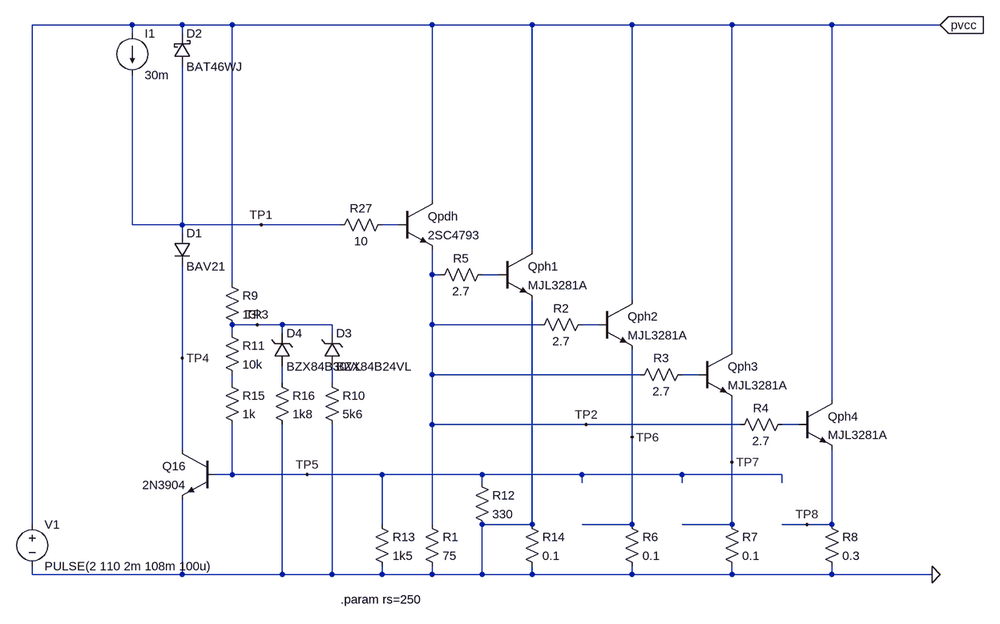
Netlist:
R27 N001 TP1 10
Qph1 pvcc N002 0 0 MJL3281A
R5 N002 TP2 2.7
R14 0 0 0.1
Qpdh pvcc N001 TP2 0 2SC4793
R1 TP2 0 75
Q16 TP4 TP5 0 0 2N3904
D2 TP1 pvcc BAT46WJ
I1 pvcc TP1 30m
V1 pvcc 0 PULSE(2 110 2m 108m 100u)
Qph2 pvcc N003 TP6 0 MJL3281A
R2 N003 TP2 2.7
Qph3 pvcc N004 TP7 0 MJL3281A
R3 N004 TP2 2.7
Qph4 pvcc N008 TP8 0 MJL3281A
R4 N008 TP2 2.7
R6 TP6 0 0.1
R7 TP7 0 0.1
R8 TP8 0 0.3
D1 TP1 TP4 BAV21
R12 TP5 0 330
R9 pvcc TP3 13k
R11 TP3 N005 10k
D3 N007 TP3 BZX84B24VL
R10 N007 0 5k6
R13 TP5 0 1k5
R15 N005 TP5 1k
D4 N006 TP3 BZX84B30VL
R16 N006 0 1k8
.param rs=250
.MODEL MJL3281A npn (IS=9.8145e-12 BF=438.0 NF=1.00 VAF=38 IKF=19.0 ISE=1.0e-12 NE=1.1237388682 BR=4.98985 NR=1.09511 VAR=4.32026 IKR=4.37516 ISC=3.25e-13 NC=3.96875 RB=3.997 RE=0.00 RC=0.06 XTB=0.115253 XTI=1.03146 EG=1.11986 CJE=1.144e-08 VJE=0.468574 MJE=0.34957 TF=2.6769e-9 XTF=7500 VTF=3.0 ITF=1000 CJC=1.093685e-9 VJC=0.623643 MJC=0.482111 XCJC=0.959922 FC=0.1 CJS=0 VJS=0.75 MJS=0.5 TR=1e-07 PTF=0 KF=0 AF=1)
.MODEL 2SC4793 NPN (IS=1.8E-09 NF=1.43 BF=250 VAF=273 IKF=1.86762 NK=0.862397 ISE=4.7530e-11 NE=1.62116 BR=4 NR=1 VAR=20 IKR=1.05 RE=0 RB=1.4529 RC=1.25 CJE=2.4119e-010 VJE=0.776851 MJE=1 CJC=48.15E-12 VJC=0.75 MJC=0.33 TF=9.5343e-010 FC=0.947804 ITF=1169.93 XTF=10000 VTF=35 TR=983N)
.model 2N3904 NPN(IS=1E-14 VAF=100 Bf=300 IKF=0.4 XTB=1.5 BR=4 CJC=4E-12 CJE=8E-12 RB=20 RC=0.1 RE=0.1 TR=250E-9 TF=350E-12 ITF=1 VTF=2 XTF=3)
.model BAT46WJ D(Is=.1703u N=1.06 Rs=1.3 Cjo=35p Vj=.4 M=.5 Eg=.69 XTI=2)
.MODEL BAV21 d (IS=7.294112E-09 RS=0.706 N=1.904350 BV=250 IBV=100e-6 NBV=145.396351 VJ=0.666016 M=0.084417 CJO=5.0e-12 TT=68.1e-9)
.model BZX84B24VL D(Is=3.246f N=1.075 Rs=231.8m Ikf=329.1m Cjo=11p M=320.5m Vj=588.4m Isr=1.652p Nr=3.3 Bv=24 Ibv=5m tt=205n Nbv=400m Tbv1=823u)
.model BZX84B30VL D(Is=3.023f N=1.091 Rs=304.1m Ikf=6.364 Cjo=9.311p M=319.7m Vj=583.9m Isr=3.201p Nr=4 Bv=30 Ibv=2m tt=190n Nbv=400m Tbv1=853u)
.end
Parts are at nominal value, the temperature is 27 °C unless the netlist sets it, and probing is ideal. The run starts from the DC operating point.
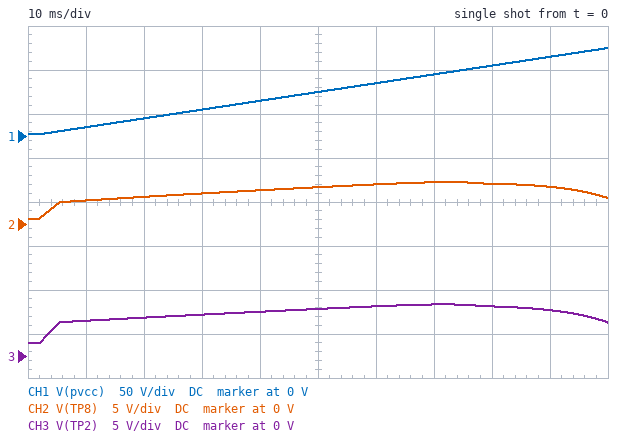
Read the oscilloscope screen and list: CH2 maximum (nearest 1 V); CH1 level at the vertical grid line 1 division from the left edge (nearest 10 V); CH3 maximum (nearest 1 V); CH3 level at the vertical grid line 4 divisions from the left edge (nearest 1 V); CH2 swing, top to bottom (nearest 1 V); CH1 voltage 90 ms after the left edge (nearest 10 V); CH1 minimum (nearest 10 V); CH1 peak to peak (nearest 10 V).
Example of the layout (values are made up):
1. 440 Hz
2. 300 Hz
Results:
1. 5 V
2. 10 V
3. 6 V
4. 5 V
5. 4 V
6. 90 V
7. 0 V
8. 100 V
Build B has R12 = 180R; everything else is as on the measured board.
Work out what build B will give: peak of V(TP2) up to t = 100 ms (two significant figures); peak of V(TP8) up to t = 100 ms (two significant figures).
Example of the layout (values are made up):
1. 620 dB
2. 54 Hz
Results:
1. 6.8 V
2. 5.8 V
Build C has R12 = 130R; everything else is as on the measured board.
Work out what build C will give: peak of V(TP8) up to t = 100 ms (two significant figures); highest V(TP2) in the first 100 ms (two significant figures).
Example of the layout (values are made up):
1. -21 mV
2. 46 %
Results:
1. 5.8 V
2. 6.8 V
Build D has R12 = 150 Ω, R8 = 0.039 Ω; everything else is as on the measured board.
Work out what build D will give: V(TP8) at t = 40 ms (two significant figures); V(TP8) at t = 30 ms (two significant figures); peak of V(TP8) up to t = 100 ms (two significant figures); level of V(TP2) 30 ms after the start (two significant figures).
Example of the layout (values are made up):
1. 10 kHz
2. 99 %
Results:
1. 1.5 V
2. 1.3 V
3. 2.9 V
4. 4.0 V
